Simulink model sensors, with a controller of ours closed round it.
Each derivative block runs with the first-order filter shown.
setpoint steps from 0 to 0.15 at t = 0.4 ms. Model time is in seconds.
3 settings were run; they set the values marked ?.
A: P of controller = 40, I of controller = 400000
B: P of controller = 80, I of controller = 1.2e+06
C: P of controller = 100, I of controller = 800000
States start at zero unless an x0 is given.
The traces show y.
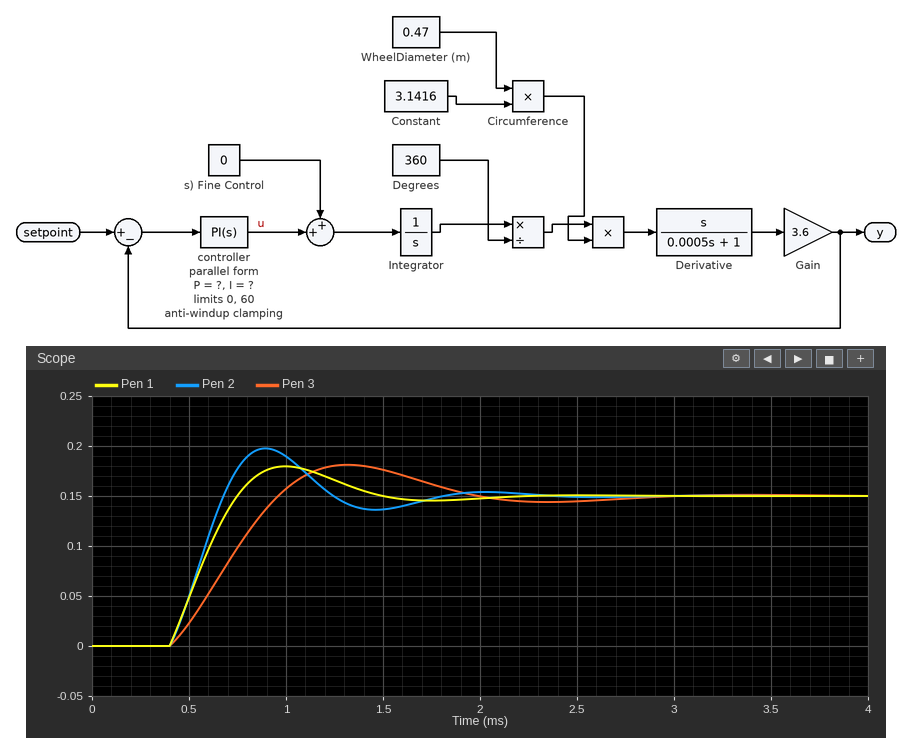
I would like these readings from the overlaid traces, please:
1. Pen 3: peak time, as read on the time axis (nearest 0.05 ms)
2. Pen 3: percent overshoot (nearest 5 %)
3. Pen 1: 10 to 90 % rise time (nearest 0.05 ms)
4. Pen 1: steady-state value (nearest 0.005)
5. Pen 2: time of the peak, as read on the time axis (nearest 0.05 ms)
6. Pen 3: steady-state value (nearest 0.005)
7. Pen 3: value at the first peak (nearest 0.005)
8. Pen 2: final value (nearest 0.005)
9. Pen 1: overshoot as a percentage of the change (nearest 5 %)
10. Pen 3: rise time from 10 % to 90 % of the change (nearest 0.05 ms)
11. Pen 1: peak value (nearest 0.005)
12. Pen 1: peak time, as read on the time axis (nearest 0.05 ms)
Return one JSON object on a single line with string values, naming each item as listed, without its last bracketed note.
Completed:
{"Pen 3: peak time, as read on the time axis": "1.30 ms", "Pen 3: percent overshoot": "20 %", "Pen 1: 10 to 90 % rise time": "0.25 ms", "Pen 1: steady-state value": "0.150", "Pen 2: time of the peak, as read on the time axis": "0.90 ms", "Pen 3: steady-state value": "0.150", "Pen 3: value at the first peak": "0.180", "Pen 2: final value": "0.150", "Pen 1: overshoot as a percentage of the change": "20 %", "Pen 3: rise time from 10 % to 90 % of the change": "0.40 ms", "Pen 1: peak value": "0.180", "Pen 1: peak time, as read on the time axis": "1.00 ms"}
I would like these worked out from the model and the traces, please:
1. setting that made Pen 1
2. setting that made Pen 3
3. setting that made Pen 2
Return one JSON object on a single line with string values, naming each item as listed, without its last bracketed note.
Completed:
{"setting that made Pen 1": "C", "setting that made Pen 3": "A", "setting that made Pen 2": "B"}
